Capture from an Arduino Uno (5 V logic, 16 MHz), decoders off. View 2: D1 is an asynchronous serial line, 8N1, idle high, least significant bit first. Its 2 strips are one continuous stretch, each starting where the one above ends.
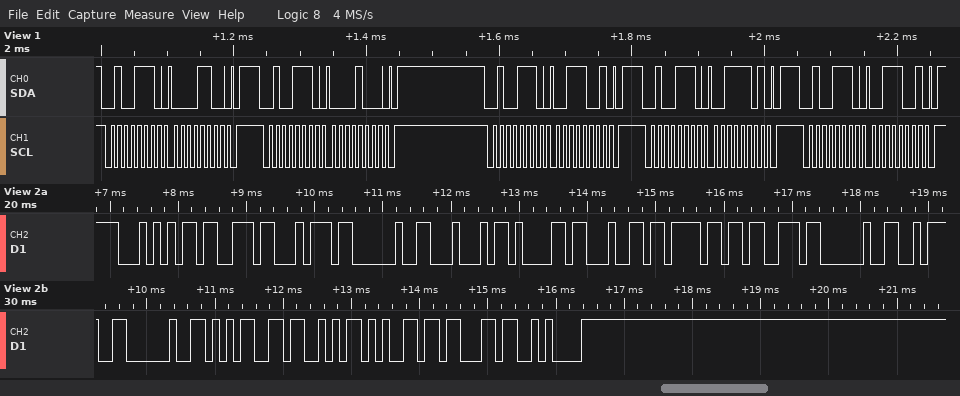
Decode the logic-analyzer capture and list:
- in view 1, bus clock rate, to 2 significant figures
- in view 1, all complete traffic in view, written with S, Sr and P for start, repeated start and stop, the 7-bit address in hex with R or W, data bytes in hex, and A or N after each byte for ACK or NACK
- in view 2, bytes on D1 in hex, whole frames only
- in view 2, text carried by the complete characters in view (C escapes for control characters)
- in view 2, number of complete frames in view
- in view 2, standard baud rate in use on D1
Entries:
100 kHz
S 27W A 0C A P S 27W A 08 A P S 27W A 39 A P S 27W A 3D A P S 27W A 39 A P
54 73 74 20 44 61 64 6F 73 20 3A 20 35 53 65 63 0A
"Tst Dados : 5Sec\n"
17
9600 baud
